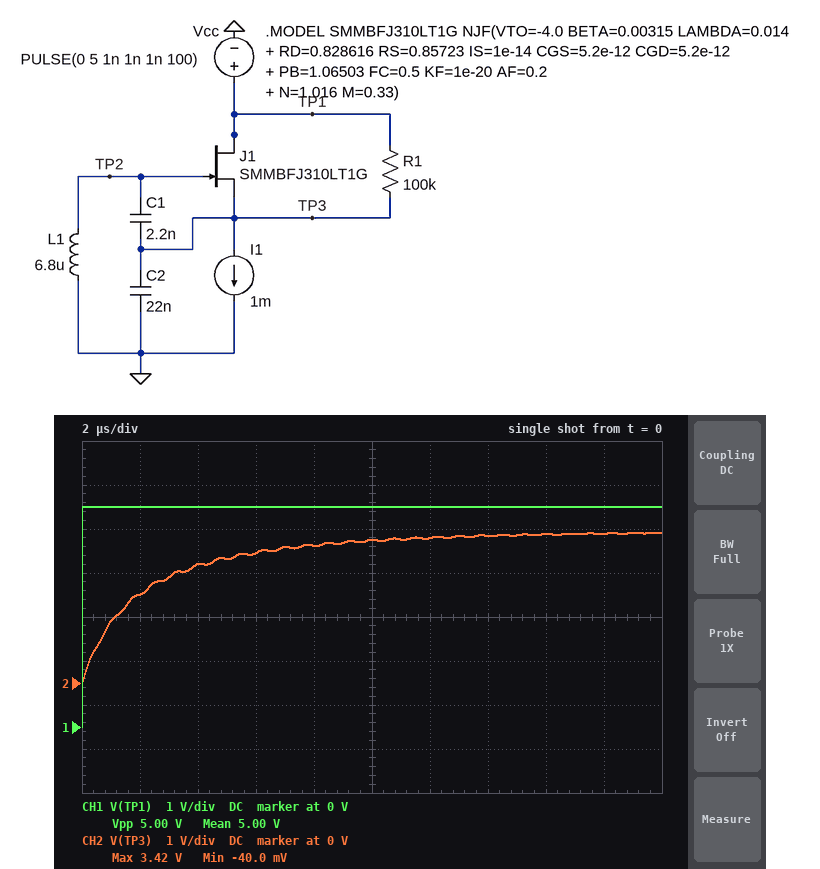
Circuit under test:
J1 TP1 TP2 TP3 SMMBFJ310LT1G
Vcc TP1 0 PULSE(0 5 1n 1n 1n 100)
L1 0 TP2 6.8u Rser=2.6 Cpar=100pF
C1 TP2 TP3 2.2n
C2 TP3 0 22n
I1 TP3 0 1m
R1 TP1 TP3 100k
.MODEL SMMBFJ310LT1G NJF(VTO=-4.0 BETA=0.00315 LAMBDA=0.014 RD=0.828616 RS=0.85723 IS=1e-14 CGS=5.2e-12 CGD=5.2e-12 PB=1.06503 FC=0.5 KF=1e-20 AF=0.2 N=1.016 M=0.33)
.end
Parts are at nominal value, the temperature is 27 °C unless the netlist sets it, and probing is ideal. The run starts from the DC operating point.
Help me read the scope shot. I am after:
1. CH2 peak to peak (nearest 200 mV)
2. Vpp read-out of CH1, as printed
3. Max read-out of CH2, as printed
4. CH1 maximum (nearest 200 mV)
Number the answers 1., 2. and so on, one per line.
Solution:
1. 3.4 V
2. 5.00 V
3. 3.42 V
4. 5.0 V
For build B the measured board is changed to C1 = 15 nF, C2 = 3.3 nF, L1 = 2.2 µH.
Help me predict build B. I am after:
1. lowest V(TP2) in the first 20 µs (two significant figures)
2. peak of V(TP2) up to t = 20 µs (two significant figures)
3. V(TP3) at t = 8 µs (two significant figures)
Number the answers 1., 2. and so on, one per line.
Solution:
1. -1.2 V
2. 1.2 V
3. 3.3 V
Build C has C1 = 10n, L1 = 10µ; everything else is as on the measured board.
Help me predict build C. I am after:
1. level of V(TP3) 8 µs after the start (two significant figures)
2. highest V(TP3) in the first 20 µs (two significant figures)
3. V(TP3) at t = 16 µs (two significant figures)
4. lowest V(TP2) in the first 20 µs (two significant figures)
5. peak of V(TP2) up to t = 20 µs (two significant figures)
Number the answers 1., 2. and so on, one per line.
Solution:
1. 2.8 V
2. 3.5 V
3. 3.2 V
4. -900 mV
5. 900 mV
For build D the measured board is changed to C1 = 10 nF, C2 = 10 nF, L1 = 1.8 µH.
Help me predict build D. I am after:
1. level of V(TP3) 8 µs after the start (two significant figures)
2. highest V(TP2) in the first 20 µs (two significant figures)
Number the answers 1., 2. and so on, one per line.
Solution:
1. 3.2 V
2. 490 mV
